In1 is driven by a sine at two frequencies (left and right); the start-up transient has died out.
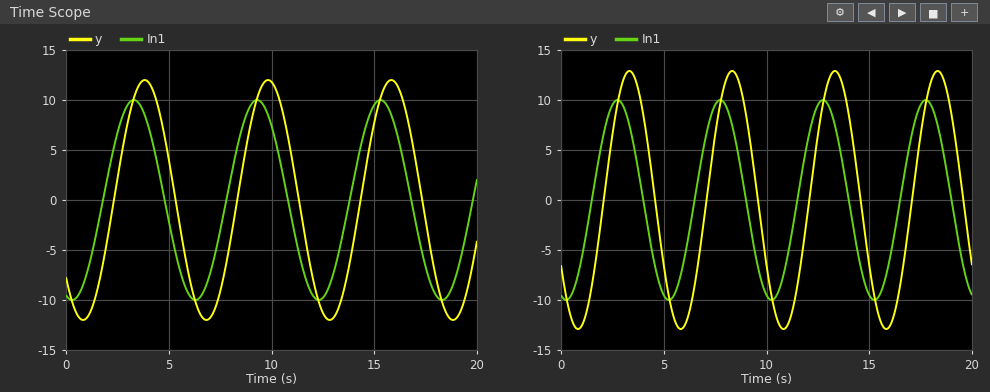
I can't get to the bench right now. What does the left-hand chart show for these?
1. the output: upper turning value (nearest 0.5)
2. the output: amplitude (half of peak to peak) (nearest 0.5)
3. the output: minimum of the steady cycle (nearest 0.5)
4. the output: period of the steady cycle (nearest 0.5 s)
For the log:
12.0
12.0
-12.0
6.0 s
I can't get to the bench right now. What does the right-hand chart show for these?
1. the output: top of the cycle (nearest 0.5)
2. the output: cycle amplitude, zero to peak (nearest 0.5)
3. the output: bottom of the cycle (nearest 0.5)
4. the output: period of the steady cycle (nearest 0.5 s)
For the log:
13.0
13.0
-13.0
5.0 s
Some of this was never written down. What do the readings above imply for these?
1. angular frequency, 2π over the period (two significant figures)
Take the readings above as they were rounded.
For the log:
1.3 rad/s
